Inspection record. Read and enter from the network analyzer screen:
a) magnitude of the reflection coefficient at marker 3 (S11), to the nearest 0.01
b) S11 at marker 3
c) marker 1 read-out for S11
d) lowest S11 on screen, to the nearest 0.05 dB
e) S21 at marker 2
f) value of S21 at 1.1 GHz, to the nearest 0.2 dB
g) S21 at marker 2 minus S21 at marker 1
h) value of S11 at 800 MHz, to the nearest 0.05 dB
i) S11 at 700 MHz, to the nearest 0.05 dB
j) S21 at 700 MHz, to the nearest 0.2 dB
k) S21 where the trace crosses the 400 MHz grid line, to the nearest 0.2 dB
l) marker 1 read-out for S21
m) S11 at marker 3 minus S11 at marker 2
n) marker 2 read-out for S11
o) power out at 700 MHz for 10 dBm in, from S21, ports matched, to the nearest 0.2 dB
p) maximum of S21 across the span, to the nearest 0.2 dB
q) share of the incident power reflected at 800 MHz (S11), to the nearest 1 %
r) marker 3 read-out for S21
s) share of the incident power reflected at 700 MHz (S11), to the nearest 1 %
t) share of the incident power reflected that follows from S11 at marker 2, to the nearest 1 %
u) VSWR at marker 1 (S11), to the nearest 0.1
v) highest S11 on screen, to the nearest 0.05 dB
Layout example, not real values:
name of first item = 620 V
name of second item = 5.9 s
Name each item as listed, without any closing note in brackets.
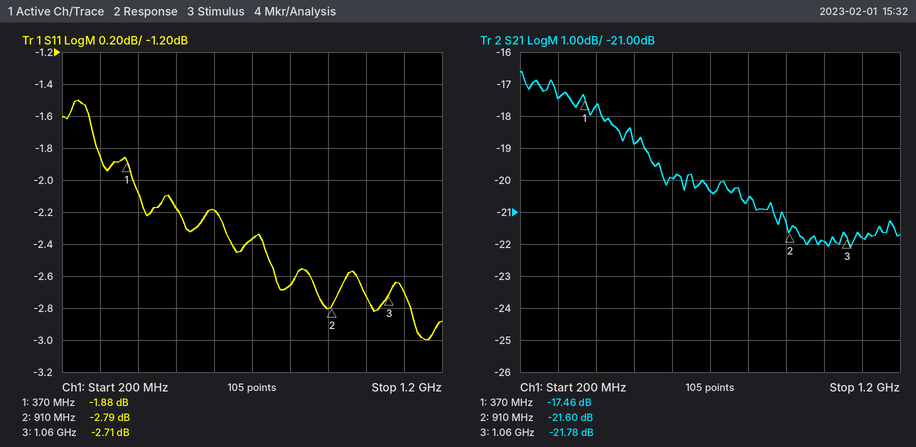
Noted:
magnitude of the reflection coefficient at marker 3 (S11), to the nearest 0.01 = 0.73
S11 at marker 3 = -2.71 dB
marker 1 read-out for S11 = -1.88 dB
lowest S11 on screen, to the nearest 0.05 dB = -3.00 dB
S21 at marker 2 = -21.60 dB
value of S21 at 1.1 GHz, to the nearest 0.2 dB = -21.8 dB
S21 at marker 2 minus S21 at marker 1 = -4.14 dB
value of S11 at 800 MHz, to the nearest 0.05 dB = -2.65 dB
S11 at 700 MHz, to the nearest 0.05 dB = -2.35 dB
S21 at 700 MHz, to the nearest 0.2 dB = -20.4 dB
S21 where the trace crosses the 400 MHz grid line, to the nearest 0.2 dB = -17.6 dB
marker 1 read-out for S21 = -17.46 dB
S11 at marker 3 minus S11 at marker 2 = 0.08 dB
marker 2 read-out for S11 = -2.79 dB
power out at 700 MHz for 10 dBm in, from S21, ports matched, to the nearest 0.2 dB = -10.4 dBm
maximum of S21 across the span, to the nearest 0.2 dB = -16.6 dB
share of the incident power reflected at 800 MHz (S11), to the nearest 1 % = 54 %
marker 3 read-out for S21 = -21.78 dB
share of the incident power reflected at 700 MHz (S11), to the nearest 1 % = 58 %
share of the incident power reflected that follows from S11 at marker 2, to the nearest 1 % = 53 %
VSWR at marker 1 (S11), to the nearest 0.1 = 9.3
highest S11 on screen, to the nearest 0.05 dB = -1.50 dB
